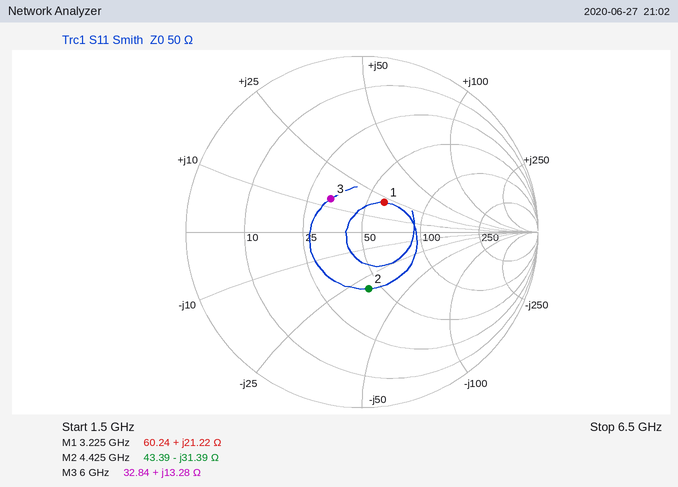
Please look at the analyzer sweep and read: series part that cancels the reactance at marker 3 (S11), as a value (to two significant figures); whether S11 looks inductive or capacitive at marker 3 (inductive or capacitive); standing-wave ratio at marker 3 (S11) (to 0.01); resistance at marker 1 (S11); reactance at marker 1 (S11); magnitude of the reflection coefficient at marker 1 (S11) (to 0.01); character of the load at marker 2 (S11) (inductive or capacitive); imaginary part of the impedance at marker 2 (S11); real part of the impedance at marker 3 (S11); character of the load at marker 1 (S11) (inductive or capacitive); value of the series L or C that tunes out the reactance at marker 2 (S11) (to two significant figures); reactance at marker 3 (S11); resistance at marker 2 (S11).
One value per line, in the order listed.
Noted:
2.0 pF
inductive
1.70
60.24 Ω
+21.22 Ω
0.21
capacitive
-31.39 Ω
32.84 Ω
inductive
1.1 nH
+13.28 Ω
43.39 Ω
